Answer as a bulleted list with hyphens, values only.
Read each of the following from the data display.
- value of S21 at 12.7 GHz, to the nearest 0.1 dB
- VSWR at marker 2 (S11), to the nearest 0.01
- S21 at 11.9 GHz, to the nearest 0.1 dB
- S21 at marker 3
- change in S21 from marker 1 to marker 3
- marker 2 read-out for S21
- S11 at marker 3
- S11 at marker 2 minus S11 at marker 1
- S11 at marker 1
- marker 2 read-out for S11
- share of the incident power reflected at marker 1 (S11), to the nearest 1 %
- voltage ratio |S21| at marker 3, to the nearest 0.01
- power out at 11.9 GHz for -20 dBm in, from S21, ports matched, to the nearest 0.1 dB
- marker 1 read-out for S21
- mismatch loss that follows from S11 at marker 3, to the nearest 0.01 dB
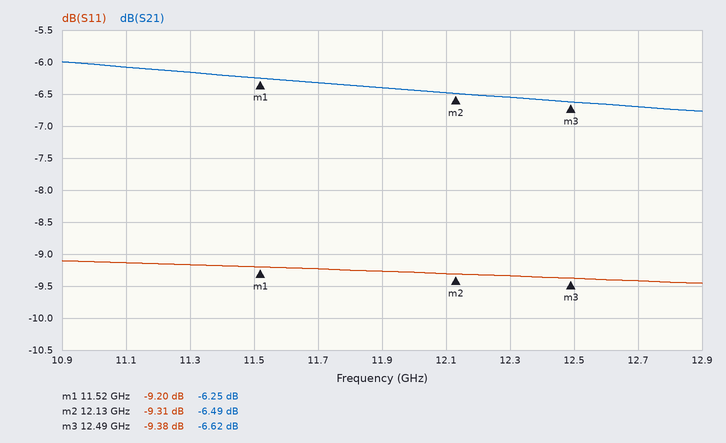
- -6.7 dB
- 2.04
- -6.4 dB
- -6.62 dB
- -0.37 dB
- -6.49 dB
- -9.38 dB
- -0.11 dB
- -9.20 dB
- -9.31 dB
- 12 %
- 0.47
- -26.4 dBm
- -6.25 dB
- 0.53 dB
